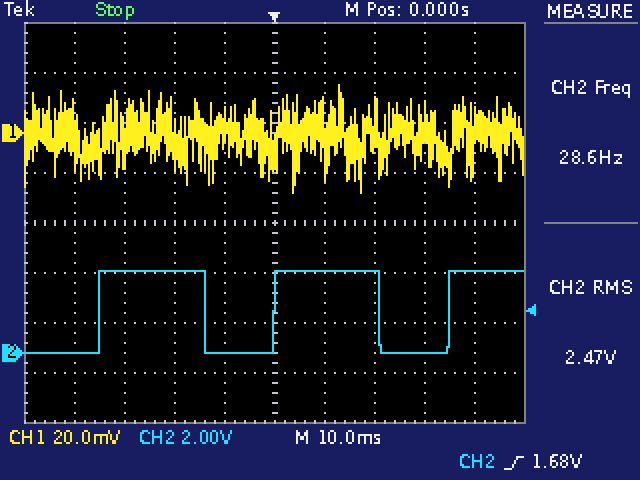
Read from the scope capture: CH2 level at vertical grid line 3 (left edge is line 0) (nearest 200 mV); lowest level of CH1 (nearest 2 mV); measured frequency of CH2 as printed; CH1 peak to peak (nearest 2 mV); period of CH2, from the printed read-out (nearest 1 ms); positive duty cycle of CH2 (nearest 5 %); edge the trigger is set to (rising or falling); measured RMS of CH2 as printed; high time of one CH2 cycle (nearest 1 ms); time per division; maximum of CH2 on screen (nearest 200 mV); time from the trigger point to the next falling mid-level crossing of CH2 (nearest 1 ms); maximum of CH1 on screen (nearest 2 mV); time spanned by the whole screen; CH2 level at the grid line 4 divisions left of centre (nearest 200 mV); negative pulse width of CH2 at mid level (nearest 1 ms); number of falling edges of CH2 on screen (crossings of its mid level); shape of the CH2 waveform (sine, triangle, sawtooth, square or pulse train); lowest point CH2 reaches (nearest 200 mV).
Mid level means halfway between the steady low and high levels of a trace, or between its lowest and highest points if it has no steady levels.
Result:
3.2 V
-24 mV
28.6 Hz
44 mV
35 ms
60 %
rising
2.47 V
21 ms
10 ms
3.2 V
21 ms
20 mV
100 ms
0.0 V
14 ms
2
pulse train
0.0 V
